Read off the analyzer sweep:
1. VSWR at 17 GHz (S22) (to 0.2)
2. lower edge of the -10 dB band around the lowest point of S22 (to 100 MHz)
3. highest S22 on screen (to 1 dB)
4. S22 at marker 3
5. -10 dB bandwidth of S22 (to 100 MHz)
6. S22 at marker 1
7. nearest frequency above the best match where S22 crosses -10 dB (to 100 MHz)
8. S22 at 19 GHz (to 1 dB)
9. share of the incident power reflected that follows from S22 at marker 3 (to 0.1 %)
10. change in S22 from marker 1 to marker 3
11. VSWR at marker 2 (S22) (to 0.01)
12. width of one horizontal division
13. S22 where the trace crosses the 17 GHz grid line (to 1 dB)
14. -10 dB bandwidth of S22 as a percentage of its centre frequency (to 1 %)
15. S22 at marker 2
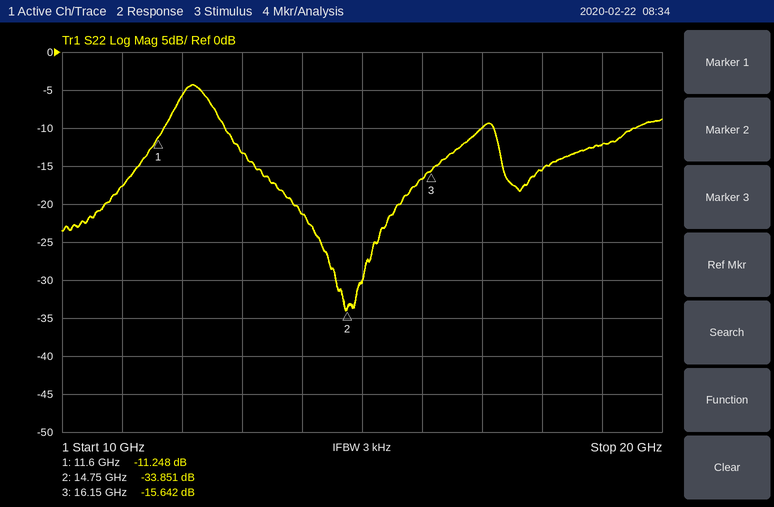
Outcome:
2.0
12.7 GHz
-4 dB
-15.642 dB
4.3 GHz
-11.248 dB
17.0 GHz
-12 dB
2.7 %
-4.394 dB
1.04
1 GHz
-10 dB
29 %
-33.851 dB
